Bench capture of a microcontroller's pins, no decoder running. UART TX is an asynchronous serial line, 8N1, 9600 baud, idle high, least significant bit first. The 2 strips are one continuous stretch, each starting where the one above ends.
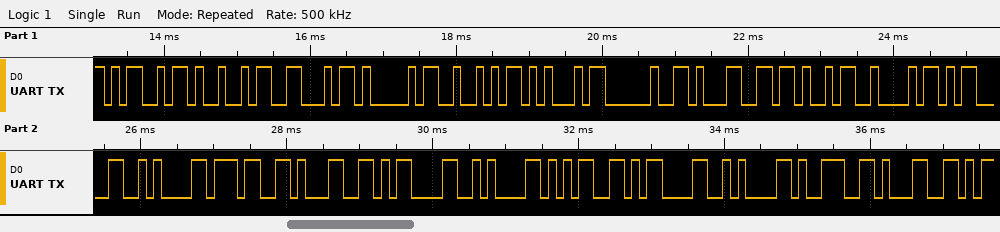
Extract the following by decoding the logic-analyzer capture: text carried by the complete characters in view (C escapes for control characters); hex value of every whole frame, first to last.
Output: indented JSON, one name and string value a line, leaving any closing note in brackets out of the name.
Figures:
{
  "text carried by the complete characters in view": "\"MIFARE 1KB\\r\\n71\\r\\n5\\r\\n91\"",
  "hex value of every whole frame, first to last": "4D 49 46 41 52 45 20 31 4B 42 0D 0A 37 31 0D 0A 35 0D 0A 39 31"
}
